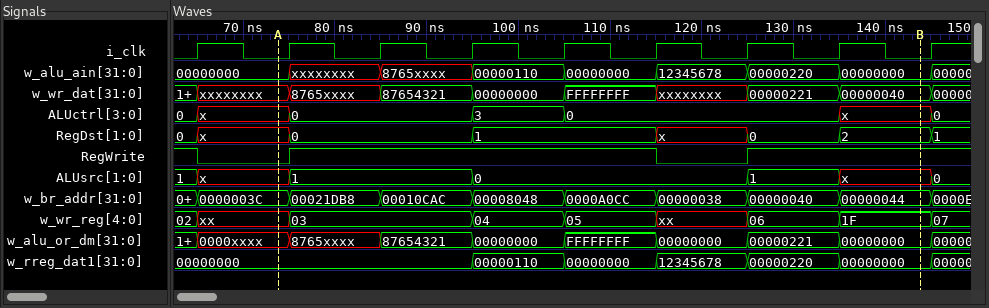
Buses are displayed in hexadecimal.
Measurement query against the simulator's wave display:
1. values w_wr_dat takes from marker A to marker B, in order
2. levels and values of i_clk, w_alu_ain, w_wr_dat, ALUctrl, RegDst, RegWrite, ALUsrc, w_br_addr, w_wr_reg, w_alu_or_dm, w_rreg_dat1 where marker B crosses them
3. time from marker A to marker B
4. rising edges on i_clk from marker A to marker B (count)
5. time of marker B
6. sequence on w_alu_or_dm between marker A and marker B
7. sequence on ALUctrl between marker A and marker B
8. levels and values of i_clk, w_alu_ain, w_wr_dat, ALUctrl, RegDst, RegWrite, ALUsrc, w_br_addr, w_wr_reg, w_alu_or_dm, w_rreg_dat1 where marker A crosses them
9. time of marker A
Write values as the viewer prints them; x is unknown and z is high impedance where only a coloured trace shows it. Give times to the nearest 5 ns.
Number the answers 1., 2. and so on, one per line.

1. xxxxxxxx, 8765xxxx, 87654321, 00000000, FFFFFFFF, xxxxxxxx, 00000221, 00000040
2. i_clk=0, w_alu_ain=00000000, w_wr_dat=00000040, ALUctrl=x, RegDst=2, RegWrite=1, ALUsrc=x, w_br_addr=00000044, w_wr_reg=1F, w_alu_or_dm=00000000, w_rreg_dat1=00000000
3. 70 ns
4. 7
5. 145 ns
6. 0000xxxx, 8765xxxx, 87654321, 00000000, FFFFFFFF, 00000000, 00000221, 00000000
7. x, 0, 3, 0, x
8. i_clk=0, w_alu_ain=00000000, w_wr_dat=xxxxxxxx, ALUctrl=x, RegDst=x, RegWrite=0, ALUsrc=x, w_br_addr=0000003C, w_wr_reg=xx, w_alu_or_dm=0000xxxx, w_rreg_dat1=00000000
9. 75 ns
